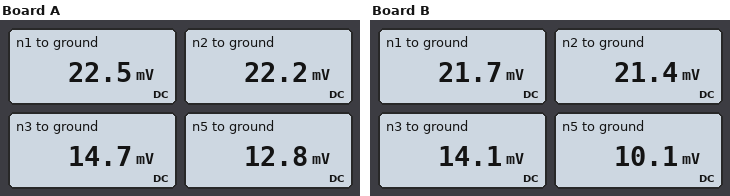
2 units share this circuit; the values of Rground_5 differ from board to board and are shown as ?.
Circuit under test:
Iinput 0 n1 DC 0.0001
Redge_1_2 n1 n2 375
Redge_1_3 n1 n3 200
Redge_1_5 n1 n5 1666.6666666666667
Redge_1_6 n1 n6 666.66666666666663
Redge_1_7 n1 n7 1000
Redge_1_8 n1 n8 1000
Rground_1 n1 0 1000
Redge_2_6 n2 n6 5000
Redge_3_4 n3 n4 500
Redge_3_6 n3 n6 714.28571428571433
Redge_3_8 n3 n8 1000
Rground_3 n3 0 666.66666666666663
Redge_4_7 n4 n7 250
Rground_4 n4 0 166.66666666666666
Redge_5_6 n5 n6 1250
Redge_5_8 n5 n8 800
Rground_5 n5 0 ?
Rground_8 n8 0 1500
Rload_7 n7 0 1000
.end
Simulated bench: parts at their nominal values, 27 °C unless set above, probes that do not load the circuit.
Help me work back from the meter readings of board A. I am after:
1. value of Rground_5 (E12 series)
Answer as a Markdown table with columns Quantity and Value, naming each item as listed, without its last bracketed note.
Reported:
| Quantity | Value |
|---|---|
| value of Rground_5 | 1.2 kΩ |
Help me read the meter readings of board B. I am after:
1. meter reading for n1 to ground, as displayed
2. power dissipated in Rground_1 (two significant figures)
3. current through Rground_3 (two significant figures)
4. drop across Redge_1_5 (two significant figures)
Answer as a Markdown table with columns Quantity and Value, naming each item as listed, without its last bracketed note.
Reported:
| Quantity | Value |
|---|---|
| meter reading for n1 to ground, as displayed | 21.7 mV |
| power dissipated in Rground_1 | 470 nW |
| current through Rground_3 | 21 µA |
| drop across Redge_1_5 | 12 mV |
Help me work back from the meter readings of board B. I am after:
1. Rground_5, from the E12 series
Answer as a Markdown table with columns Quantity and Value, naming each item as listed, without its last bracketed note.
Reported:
| Quantity | Value |
|---|---|
| Rground_5, from the E12 series | 680 Ω |
